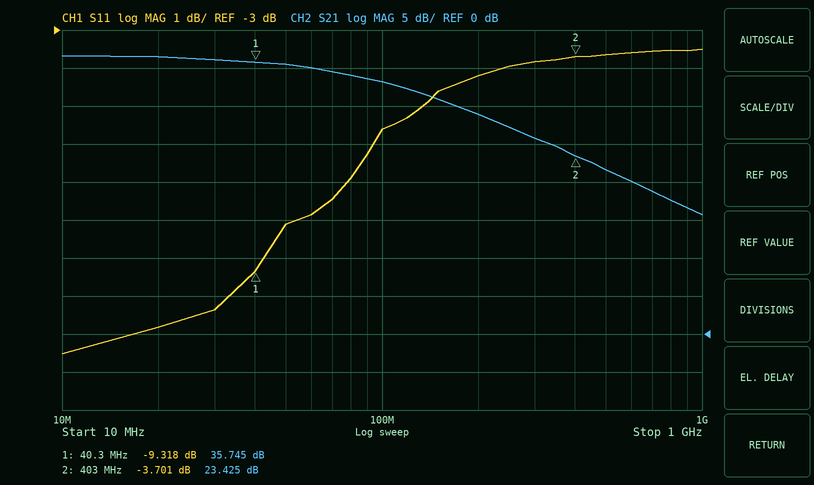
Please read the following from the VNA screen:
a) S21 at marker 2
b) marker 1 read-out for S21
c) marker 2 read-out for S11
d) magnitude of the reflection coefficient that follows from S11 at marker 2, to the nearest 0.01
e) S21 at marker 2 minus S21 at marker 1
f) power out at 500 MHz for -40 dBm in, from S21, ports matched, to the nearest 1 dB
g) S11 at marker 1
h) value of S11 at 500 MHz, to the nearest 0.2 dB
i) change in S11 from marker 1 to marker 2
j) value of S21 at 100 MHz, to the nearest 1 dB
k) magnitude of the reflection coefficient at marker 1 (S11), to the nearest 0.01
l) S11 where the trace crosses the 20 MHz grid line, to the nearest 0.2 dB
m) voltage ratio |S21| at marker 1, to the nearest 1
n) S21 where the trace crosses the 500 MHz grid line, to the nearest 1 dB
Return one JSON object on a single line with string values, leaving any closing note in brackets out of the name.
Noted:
{"S21 at marker 2": "23.425 dB", "marker 1 read-out for S21": "35.745 dB", "marker 2 read-out for S11": "-3.701 dB", "magnitude of the reflection coefficient that follows from S11 at marker 2, to the nearest 0.01": "0.65", "S21 at marker 2 minus S21 at marker 1": "-12.320 dB", "power out at 500 MHz for -40 dBm in, from S21, ports matched, to the nearest 1 dB": "-18 dBm", "S11 at marker 1": "-9.318 dB", "value of S11 at 500 MHz, to the nearest 0.2 dB": "-3.6 dB", "change in S11 from marker 1 to marker 2": "5.617 dB", "value of S21 at 100 MHz, to the nearest 1 dB": "33 dB", "magnitude of the reflection coefficient at marker 1 (S11), to the nearest 0.01": "0.34", "S11 where the trace crosses the 20 MHz grid line, to the nearest 0.2 dB": "-10.8 dB", "voltage ratio |S21| at marker 1, to the nearest 1": "61", "S21 where the trace crosses the 500 MHz grid line, to the nearest 1 dB": "22 dB"}
